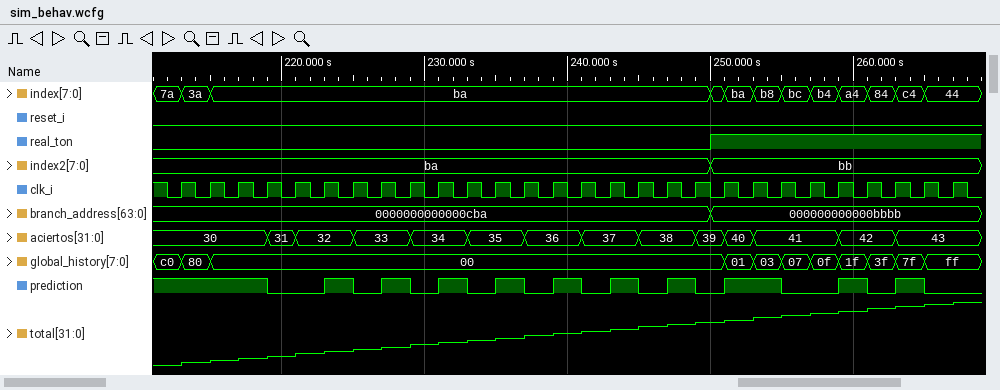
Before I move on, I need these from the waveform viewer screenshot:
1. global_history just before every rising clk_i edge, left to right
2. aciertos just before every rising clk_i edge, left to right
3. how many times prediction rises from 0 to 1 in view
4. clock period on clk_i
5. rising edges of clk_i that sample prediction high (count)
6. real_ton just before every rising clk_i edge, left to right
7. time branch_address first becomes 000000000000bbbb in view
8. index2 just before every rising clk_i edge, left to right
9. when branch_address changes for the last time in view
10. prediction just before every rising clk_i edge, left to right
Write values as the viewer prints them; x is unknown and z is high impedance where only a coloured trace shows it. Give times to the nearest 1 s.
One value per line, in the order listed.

c0, 80, 00, 00, 00, 00, 00, 00, 00, 00, 00, 00, 00, 00, 00, 00, 00, 00, 00, 00, 01, 03, 07, 0f, 1f, 3f, 7f, ff
30, 30, 30, 30, 31, 32, 32, 33, 33, 34, 34, 35, 35, 36, 36, 37, 37, 38, 38, 39, 40, 41, 41, 41, 42, 42, 43, 43
10
2 s
15
0 0 0 0 0 0 0 0 0 0 0 0 0 0 0 0 0 0 0 1 1 1 1 1 1 1 1 1
250 s
ba, ba, ba, ba, ba, ba, ba, ba, ba, ba, ba, ba, ba, ba, ba, ba, ba, ba, ba, bb, bb, bb, bb, bb, bb, bb, bb, bb
250 s
1 1 1 1 0 0 1 0 1 0 1 0 1 0 1 0 1 0 1 0 1 1 0 0 1 0 1 0
